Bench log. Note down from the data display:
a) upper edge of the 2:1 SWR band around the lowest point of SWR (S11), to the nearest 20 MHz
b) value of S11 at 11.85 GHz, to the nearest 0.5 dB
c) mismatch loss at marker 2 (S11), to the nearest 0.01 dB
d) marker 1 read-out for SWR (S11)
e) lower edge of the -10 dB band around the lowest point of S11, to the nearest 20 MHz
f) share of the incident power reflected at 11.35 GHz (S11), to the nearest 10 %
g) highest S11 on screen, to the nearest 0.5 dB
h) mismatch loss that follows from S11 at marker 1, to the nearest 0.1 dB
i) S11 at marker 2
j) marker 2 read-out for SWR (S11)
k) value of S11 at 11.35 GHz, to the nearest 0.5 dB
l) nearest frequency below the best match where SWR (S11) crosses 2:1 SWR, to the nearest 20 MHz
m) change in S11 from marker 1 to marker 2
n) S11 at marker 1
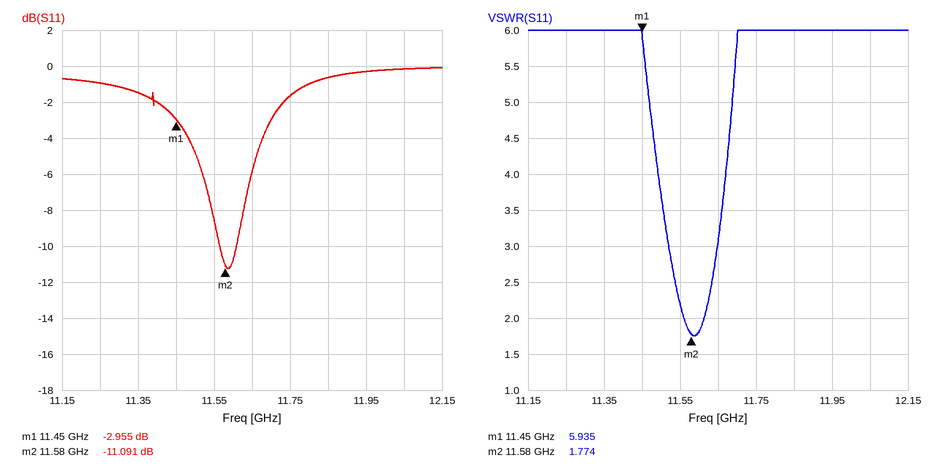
11.62 GHz
-0.5 dB
0.35 dB
5.935
11.56 GHz
70 %
0.0 dB
3.1 dB
-11.091 dB
1.774
-1.5 dB
11.56 GHz
-8.136 dB
-2.955 dB
